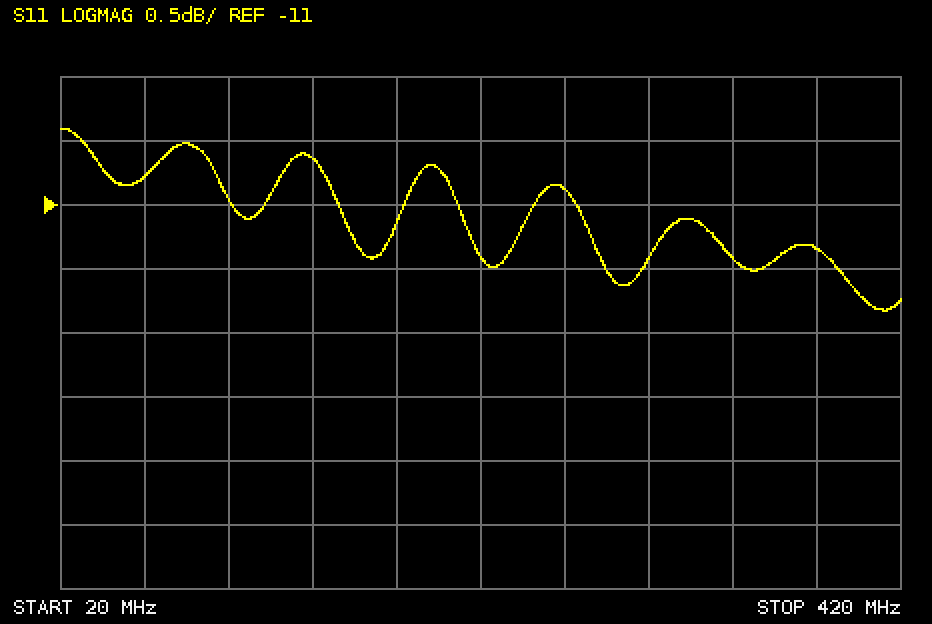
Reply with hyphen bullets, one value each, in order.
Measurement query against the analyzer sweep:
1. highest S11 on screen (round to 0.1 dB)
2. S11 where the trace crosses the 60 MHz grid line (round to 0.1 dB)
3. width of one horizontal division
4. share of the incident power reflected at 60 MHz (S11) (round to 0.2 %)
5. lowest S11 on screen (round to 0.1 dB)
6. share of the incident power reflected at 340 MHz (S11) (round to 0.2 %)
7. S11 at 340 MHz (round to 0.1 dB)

- -10.4 dB
- -10.8 dB
- 40 MHz
- 8.4 %
- -11.8 dB
- 7.2 %
- -11.4 dB
